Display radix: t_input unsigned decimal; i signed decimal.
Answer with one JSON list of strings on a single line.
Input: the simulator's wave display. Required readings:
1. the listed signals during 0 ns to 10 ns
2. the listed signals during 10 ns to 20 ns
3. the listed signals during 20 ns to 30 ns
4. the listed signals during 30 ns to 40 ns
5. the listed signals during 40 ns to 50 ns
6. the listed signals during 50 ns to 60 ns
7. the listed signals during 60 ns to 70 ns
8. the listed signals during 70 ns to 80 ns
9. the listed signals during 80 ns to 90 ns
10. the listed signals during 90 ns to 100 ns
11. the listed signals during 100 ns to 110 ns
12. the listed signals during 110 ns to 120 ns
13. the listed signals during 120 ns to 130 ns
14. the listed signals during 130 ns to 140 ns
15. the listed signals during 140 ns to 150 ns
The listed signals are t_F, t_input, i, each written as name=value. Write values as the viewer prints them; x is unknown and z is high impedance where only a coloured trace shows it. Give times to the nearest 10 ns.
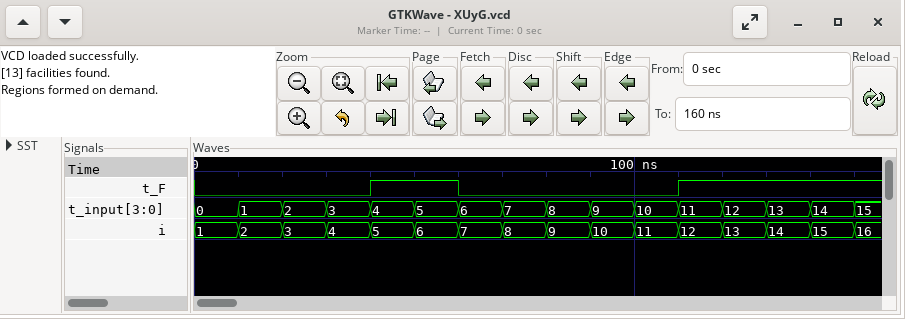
["t_F=0, t_input=0, i=1", "t_F=0, t_input=1, i=2", "t_F=0, t_input=2, i=3", "t_F=0, t_input=3, i=4", "t_F=1, t_input=4, i=5", "t_F=1, t_input=5, i=6", "t_F=0, t_input=6, i=7", "t_F=0, t_input=7, i=8", "t_F=0, t_input=8, i=9", "t_F=0, t_input=9, i=10", "t_F=0, t_input=10, i=11", "t_F=1, t_input=11, i=12", "t_F=1, t_input=12, i=13", "t_F=1, t_input=13, i=14", "t_F=1, t_input=14, i=15"]
